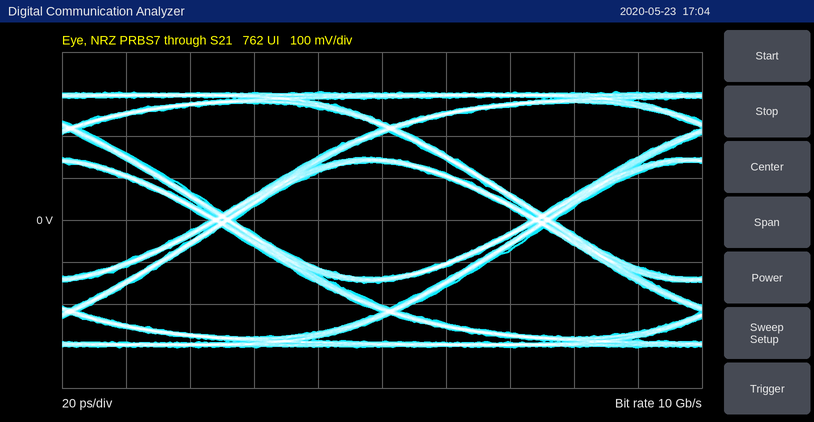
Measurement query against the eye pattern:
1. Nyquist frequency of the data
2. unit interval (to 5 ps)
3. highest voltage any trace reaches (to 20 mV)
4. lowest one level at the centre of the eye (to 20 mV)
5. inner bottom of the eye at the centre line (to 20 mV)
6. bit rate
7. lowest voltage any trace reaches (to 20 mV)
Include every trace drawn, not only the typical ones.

5 GHz
100 ps
300 mV
140 mV
-140 mV
10 Gb/s
-300 mV
